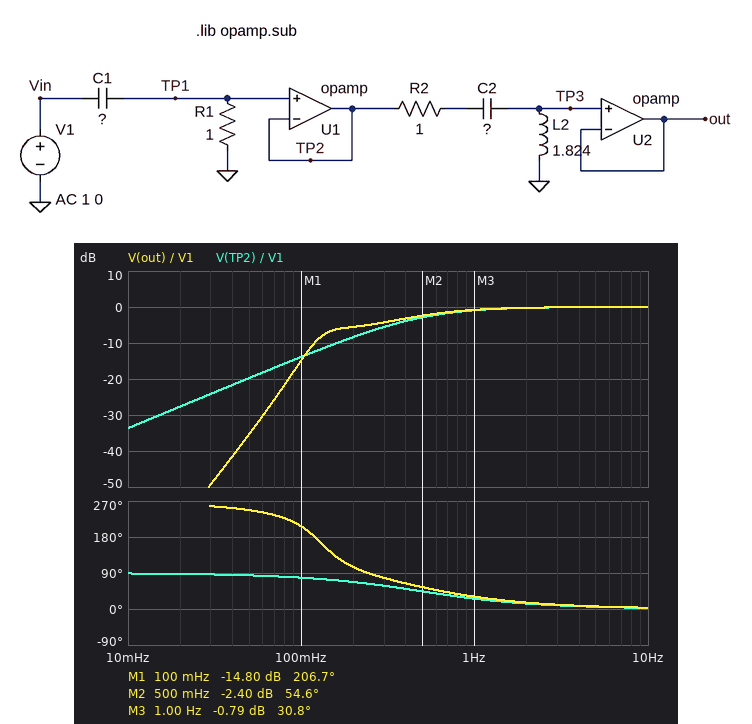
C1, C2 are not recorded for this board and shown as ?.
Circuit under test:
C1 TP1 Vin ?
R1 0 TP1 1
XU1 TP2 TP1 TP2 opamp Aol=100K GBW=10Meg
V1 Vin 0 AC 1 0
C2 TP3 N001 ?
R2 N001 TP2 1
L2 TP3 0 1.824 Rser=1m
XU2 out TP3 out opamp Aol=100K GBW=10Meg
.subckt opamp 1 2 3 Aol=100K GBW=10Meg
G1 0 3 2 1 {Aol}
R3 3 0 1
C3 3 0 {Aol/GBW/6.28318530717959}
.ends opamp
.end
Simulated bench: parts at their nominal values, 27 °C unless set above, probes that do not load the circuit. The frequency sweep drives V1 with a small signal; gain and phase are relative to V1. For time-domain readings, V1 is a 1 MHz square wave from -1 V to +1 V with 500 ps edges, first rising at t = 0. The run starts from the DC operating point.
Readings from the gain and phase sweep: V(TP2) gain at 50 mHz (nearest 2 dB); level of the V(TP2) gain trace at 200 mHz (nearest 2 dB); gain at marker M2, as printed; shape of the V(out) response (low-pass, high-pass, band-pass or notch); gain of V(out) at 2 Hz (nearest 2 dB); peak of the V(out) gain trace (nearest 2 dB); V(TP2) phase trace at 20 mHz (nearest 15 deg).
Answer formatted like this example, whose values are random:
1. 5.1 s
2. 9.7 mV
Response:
1. -20 dB
2. -8 dB
3. -2.40 dB
4. high-pass
5. 0 dB
6. 0 dB
7. 90 deg
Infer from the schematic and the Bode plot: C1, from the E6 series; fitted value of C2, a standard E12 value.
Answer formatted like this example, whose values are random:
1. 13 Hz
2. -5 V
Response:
1. 330 mF
2. 820 mF
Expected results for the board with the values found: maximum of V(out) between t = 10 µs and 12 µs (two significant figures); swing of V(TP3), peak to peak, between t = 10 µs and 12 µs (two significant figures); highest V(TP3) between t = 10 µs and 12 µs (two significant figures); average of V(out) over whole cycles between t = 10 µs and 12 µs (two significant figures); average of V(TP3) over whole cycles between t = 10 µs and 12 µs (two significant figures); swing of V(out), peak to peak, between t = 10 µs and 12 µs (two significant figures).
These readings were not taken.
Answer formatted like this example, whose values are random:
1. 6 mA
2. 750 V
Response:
1. 2.0 V
2. 2.0 V
3. 2.0 V
4. 1.0 V
5. 1.0 V
6. 2.0 V
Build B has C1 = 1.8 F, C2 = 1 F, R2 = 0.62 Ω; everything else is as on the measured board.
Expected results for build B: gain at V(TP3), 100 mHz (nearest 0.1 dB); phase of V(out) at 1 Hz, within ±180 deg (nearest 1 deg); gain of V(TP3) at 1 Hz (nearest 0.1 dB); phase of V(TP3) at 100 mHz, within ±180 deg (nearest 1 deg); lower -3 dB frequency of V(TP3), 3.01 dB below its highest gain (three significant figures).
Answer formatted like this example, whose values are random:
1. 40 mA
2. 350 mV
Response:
1. 1.0 dB
2. 8 deg
3. 0.1 dB
4. 167 deg
5. 104 mHz
